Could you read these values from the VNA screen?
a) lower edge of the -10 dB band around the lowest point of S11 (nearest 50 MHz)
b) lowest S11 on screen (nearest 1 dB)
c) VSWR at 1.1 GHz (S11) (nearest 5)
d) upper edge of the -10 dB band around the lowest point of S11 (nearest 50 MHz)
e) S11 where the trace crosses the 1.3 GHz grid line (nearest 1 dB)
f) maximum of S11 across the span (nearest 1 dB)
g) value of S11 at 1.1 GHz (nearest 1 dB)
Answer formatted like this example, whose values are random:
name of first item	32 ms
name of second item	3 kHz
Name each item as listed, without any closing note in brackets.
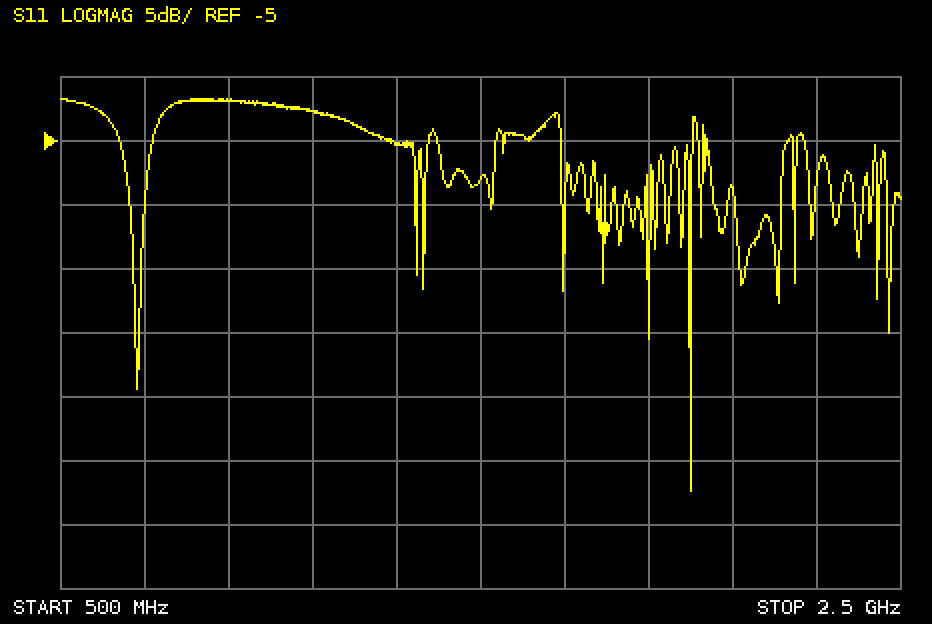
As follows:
lower edge of the -10 dB band around the lowest point of S11	2.00 GHz
lowest S11 on screen	-32 dB
VSWR at 1.1 GHz (S11)	5
upper edge of the -10 dB band around the lowest point of S11	2.00 GHz
S11 where the trace crosses the 1.3 GHz grid line	-5 dB
maximum of S11 across the span	-2 dB
value of S11 at 1.1 GHz	-3 dB
